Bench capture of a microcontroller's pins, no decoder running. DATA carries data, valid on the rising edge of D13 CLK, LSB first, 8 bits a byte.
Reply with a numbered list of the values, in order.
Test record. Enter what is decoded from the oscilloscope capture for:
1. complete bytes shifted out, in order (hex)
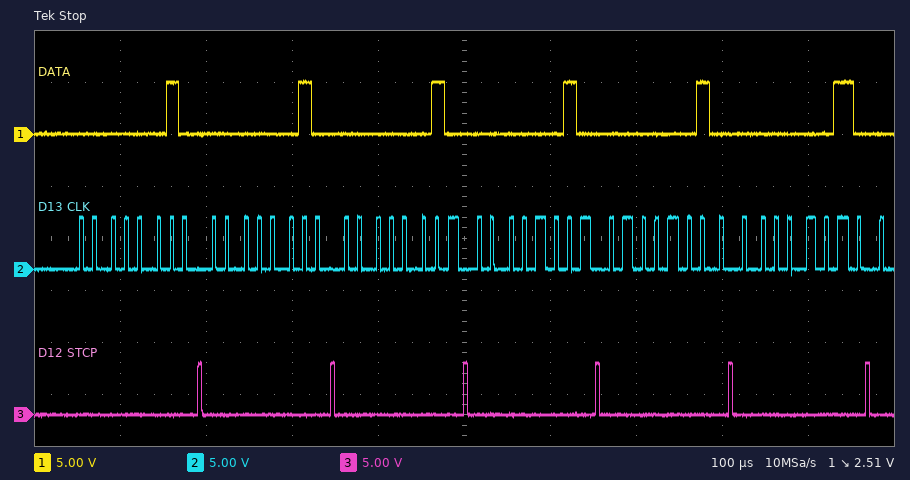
1. 0x40 0x40 0x40 0x40 0x40 0x40
